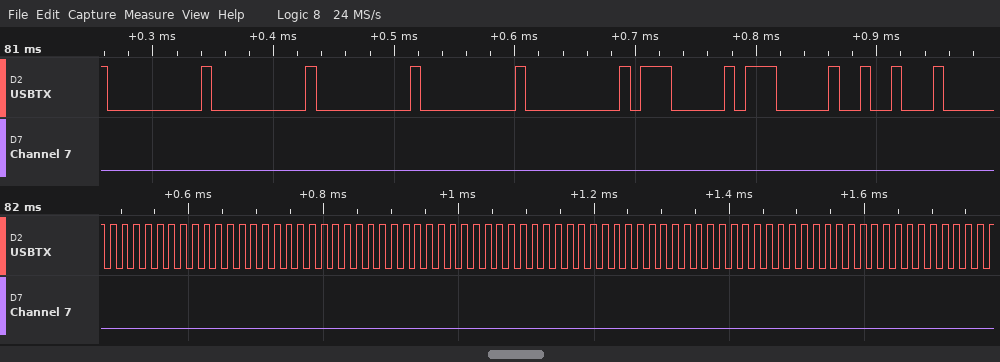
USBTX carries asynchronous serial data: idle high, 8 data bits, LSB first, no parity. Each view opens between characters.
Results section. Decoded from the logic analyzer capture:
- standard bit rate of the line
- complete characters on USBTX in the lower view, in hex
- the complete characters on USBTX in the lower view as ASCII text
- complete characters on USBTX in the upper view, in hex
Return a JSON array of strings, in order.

["115200 baud", "55, 55, 55, 55, 55, 55, 55, 55, 55, 55, 55, 55, 55, 55, 55", "\"UUUUUUUUUUUUUUU\"", "00, 00, 00, 00, 00, 07, 07, 12"]
